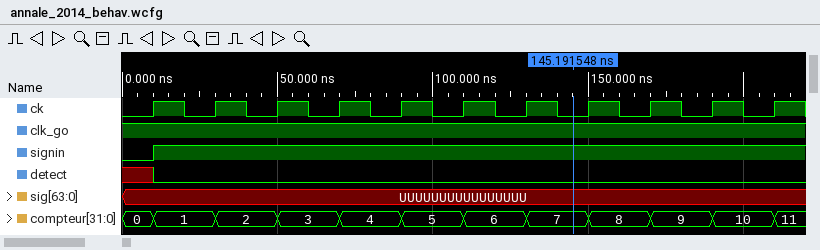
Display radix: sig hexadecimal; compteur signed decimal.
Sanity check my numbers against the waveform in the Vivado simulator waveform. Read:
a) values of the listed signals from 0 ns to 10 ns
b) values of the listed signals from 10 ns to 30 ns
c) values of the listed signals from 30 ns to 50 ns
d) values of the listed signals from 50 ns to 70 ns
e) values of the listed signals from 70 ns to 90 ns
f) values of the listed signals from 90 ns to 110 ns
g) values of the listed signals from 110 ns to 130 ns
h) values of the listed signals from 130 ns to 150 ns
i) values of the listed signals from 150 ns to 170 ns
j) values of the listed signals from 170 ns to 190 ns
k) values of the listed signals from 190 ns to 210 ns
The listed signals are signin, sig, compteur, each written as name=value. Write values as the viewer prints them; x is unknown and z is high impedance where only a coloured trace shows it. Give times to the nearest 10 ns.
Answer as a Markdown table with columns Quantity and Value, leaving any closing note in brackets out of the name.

| Quantity | Value |
|---|---|
| values of the listed signals from 0 ns to 10 ns | signin=0, sig=UUUUUUUUUUUUUUUU, compteur=0 |
| values of the listed signals from 10 ns to 30 ns | signin=1, sig=UUUUUUUUUUUUUUUU, compteur=1 |
| values of the listed signals from 30 ns to 50 ns | signin=1, sig=UUUUUUUUUUUUUUUU, compteur=2 |
| values of the listed signals from 50 ns to 70 ns | signin=1, sig=UUUUUUUUUUUUUUUU, compteur=3 |
| values of the listed signals from 70 ns to 90 ns | signin=1, sig=UUUUUUUUUUUUUUUU, compteur=4 |
| values of the listed signals from 90 ns to 110 ns | signin=1, sig=UUUUUUUUUUUUUUUU, compteur=5 |
| values of the listed signals from 110 ns to 130 ns | signin=1, sig=UUUUUUUUUUUUUUUU, compteur=6 |
| values of the listed signals from 130 ns to 150 ns | signin=1, sig=UUUUUUUUUUUUUUUU, compteur=7 |
| values of the listed signals from 150 ns to 170 ns | signin=1, sig=UUUUUUUUUUUUUUUU, compteur=8 |
| values of the listed signals from 170 ns to 190 ns | signin=1, sig=UUUUUUUUUUUUUUUU, compteur=9 |
| values of the listed signals from 190 ns to 210 ns | signin=1, sig=UUUUUUUUUUUUUUUU, compteur=10 |
